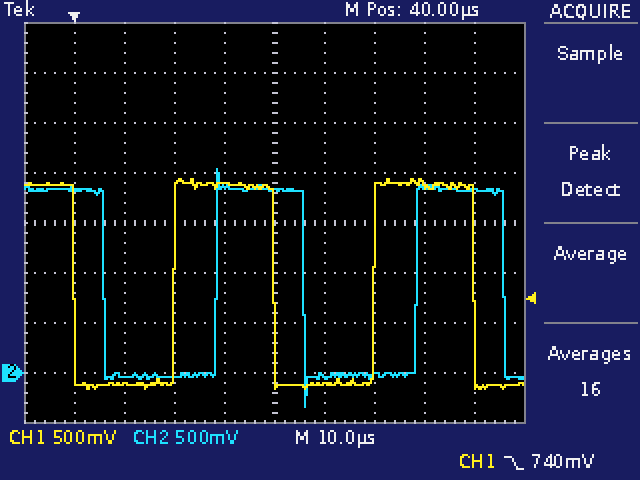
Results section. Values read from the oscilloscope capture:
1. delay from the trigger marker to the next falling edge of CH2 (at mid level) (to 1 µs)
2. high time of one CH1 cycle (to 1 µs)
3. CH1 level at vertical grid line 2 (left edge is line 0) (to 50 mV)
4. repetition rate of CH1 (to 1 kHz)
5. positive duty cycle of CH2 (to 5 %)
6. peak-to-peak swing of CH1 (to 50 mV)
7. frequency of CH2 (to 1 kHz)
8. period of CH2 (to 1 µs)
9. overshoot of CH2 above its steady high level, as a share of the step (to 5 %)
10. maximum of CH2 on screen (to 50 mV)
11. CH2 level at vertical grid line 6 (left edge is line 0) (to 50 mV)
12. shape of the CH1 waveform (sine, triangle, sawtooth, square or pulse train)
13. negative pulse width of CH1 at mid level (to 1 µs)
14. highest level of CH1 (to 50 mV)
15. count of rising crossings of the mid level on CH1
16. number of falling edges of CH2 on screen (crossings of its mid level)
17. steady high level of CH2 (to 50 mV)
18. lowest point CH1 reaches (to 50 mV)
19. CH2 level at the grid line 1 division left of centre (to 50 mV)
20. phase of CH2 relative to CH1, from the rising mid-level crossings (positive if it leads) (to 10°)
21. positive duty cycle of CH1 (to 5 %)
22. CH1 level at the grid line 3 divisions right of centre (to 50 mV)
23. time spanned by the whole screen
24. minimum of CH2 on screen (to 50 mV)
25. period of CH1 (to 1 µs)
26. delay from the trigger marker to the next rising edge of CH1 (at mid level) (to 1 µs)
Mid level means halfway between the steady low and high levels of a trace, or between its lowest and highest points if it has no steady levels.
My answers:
6 µs
20 µs
-100 mV
25 kHz
45 %
2.10 V
25 kHz
40 µs
10 %
2.05 V
-50 mV
square
20 µs
1.95 V
2
3
1.85 V
-150 mV
1.85 V
-80°
50 %
1.90 V
100 µs
-350 mV
40 µs
20 µs
